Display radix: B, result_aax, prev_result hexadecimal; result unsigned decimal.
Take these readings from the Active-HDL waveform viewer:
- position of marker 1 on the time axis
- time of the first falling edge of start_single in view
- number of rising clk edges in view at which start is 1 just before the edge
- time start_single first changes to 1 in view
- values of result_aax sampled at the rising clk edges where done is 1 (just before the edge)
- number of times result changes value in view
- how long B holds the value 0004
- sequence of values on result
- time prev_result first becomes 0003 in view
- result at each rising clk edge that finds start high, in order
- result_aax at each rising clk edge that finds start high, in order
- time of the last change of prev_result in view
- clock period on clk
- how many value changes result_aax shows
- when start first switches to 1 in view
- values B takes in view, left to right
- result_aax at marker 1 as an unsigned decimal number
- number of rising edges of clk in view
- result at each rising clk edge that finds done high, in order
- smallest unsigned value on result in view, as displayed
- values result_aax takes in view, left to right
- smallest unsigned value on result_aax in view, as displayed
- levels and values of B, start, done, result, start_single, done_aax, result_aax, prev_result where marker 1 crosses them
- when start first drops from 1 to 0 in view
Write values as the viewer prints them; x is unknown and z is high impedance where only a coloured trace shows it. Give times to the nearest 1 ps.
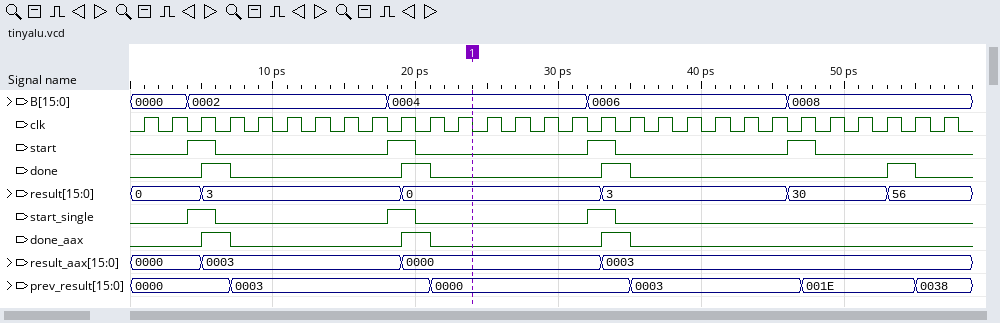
24 ps
6 ps
4
4 ps
0003, 0000, 0003, 0003
5
14 ps
0, 3, 0, 3, 30, 56
7 ps
0, 3, 0, 30
0000, 0003, 0000, 0003
55 ps
2 ps
3
4 ps
0000, 0002, 0004, 0006, 0008
0
29
3, 0, 3, 56
0
0000, 0003, 0000, 0003
0000
B=0004, start=0, done=0, result=0, start_single=0, done_aax=0, result_aax=0000, prev_result=0000
6 ps
